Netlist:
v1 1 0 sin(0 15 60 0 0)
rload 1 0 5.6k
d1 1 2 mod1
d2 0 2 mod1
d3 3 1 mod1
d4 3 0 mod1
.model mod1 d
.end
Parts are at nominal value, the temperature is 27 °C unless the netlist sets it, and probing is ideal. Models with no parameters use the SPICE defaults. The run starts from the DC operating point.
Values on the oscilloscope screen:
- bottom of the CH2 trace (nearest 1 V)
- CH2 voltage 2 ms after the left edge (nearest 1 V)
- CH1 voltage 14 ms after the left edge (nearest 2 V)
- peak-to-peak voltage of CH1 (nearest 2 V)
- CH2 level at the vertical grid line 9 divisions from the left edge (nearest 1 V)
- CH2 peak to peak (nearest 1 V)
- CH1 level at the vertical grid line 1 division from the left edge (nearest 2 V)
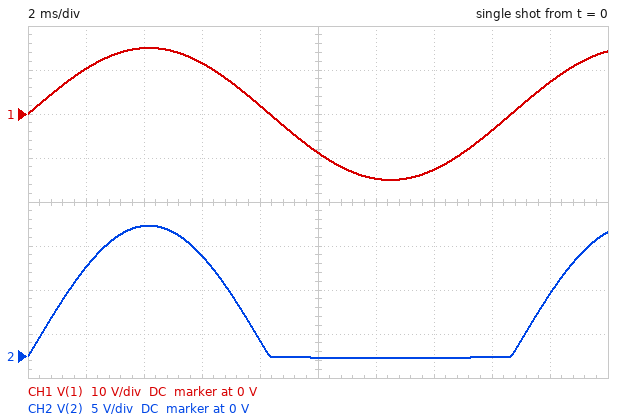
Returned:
0 V
10 V
-12 V
30 V
7 V
15 V
10 V
